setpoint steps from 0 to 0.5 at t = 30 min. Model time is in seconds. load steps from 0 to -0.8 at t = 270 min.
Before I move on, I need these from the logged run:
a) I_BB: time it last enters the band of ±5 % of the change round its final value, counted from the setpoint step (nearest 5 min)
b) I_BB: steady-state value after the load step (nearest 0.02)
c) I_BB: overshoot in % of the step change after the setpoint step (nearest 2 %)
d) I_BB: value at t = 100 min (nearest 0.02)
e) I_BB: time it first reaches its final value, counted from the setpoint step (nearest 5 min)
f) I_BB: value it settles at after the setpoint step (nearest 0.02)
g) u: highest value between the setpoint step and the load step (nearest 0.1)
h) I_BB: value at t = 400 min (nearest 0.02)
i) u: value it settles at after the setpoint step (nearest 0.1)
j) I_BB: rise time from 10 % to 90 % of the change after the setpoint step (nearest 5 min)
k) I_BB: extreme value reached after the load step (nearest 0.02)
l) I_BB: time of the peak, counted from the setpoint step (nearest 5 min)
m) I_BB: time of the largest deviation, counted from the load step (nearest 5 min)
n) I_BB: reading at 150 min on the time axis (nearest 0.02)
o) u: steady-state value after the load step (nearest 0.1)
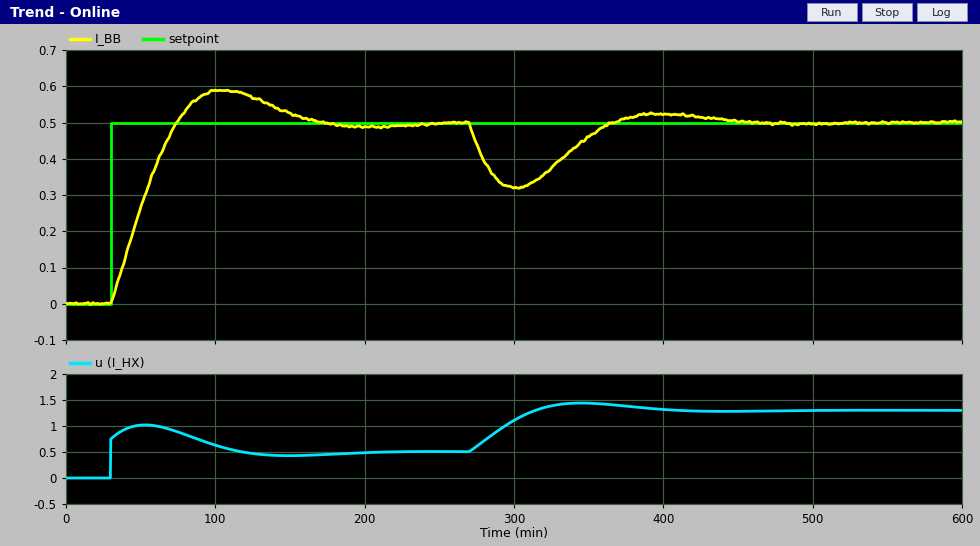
120 min
0.50
18 %
0.58
45 min
0.50
1.0
0.52
0.5
35 min
0.32
75 min
30 min
0.52
1.3
